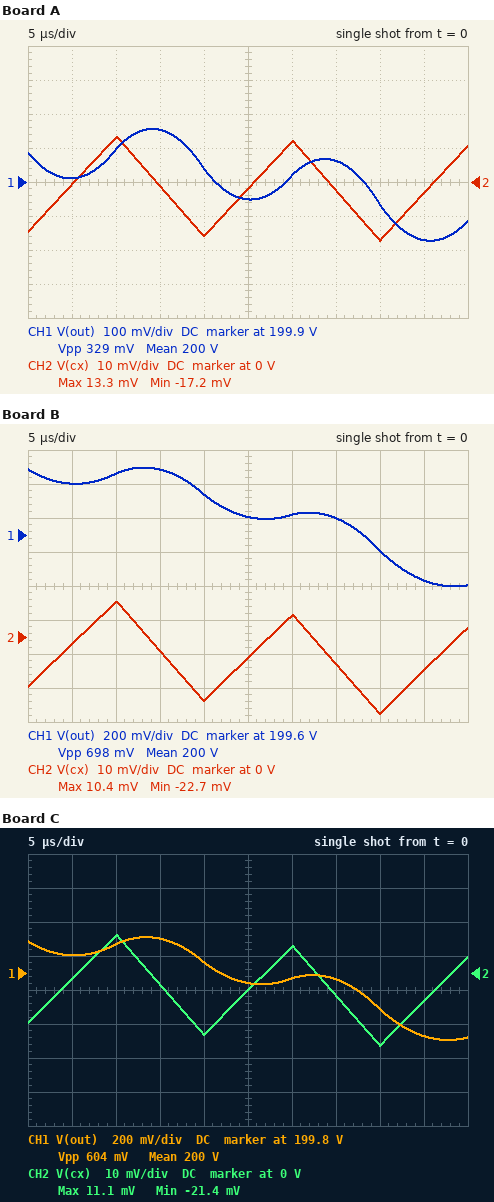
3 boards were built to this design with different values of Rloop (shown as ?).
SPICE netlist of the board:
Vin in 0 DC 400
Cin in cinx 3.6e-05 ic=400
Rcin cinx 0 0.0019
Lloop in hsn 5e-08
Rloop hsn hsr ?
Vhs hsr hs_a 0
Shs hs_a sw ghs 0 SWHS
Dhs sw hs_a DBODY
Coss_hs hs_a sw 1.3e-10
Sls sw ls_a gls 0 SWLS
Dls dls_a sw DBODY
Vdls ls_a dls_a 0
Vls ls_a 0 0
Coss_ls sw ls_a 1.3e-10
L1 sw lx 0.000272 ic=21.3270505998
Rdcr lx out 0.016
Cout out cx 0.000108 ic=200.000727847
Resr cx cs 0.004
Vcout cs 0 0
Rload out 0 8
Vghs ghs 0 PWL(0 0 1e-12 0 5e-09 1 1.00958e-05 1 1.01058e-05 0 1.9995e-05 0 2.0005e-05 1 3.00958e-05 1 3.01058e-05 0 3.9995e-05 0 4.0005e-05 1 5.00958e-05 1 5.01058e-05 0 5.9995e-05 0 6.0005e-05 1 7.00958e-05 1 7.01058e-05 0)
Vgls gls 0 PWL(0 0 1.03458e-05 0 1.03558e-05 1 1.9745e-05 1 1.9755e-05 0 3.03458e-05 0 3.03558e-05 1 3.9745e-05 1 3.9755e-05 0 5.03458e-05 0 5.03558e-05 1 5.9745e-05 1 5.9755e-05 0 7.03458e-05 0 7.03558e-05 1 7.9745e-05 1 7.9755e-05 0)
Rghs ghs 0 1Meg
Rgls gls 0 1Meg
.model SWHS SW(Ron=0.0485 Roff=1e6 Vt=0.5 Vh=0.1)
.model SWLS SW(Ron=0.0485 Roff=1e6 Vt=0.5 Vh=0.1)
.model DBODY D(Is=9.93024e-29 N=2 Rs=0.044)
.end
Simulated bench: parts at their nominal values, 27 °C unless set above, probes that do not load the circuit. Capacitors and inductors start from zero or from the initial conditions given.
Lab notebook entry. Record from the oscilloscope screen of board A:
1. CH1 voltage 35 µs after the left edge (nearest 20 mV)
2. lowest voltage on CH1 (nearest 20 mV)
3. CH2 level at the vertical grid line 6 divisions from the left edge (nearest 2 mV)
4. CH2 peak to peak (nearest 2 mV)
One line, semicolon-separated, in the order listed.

199.96 V; 199.72 V; 12 mV; 30 mV
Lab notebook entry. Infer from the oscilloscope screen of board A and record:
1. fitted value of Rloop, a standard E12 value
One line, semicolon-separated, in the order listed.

0.39 Ω
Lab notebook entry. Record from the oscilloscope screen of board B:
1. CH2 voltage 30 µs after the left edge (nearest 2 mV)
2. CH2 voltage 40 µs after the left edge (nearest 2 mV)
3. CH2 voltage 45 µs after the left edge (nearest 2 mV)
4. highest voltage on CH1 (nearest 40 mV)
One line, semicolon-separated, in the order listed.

6 mV; -22 mV; -10 mV; 200.00 V
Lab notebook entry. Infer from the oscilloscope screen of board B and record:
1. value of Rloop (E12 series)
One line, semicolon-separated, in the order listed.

1.2 Ω
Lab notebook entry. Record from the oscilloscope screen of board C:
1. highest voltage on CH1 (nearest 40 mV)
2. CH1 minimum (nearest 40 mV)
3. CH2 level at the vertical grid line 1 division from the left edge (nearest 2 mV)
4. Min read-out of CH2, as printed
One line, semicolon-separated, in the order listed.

200.00 V; 199.40 V; -2 mV; -21.4 mV
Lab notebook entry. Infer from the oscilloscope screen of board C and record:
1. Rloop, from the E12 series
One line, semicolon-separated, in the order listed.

1 Ω
